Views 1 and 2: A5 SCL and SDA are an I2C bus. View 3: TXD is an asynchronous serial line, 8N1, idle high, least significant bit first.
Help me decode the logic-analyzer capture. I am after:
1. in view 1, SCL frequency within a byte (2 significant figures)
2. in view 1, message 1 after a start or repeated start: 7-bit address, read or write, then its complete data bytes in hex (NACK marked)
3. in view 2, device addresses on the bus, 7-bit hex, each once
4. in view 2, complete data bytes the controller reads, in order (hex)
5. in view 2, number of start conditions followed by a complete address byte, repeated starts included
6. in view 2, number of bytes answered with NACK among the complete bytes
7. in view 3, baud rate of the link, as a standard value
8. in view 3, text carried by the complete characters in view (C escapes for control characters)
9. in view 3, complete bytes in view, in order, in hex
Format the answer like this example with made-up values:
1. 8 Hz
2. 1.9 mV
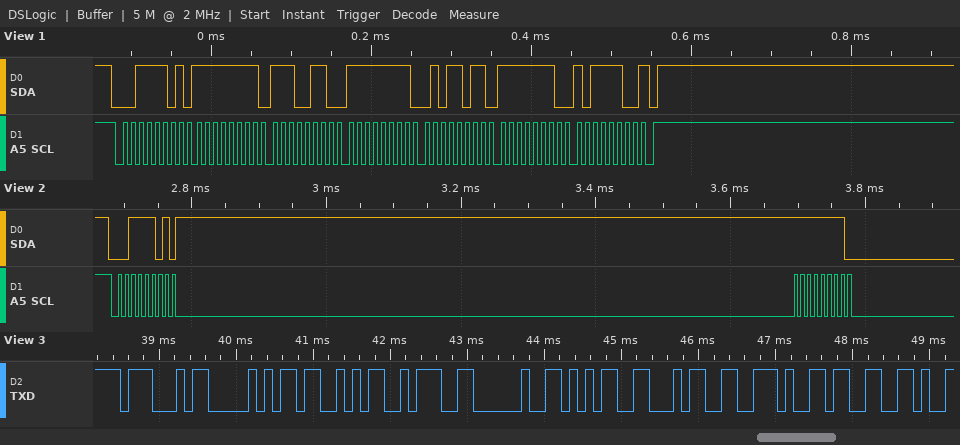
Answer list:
1. 100 kHz
2. 0x1E read: FF E6 FF 5B FE BC NACK
3. 0x1E
4. FF
5. 1
6. 0
7. 9600 baud
8. "GPS: 54.3"
9. 0x47 0x50 0x53 0x3A 0x20 0x35 0x34 0x2E 0x33
